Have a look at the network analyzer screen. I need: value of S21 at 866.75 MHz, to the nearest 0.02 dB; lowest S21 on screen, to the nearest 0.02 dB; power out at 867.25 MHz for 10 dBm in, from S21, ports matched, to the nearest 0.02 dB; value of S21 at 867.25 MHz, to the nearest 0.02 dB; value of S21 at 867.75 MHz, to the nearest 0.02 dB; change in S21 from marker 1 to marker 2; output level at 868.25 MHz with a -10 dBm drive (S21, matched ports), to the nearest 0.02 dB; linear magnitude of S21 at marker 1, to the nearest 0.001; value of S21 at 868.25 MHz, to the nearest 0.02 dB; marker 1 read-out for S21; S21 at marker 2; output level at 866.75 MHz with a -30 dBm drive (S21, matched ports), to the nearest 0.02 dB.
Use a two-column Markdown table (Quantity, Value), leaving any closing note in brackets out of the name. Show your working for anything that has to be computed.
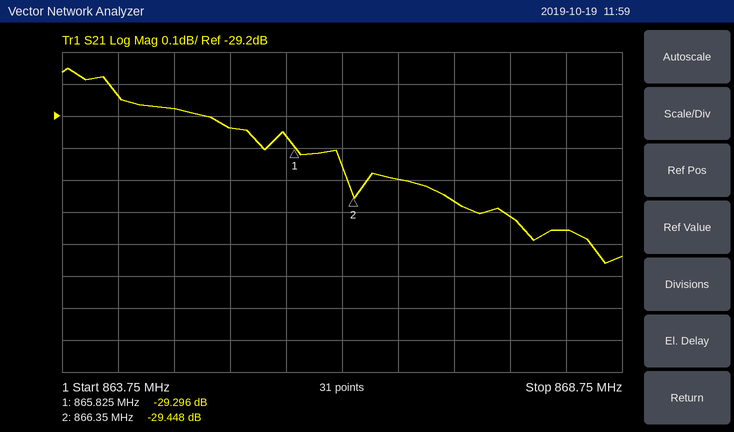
| Quantity | Value |
|---|---|
| value of S21 at 866.75 MHz, to the nearest 0.02 dB | -29.40 dB |
| lowest S21 on screen, to the nearest 0.02 dB | -29.66 dB |
| power out at 867.25 MHz for 10 dBm in, from S21, ports matched, to the nearest 0.02 dB | 10 dBm + (-29.46 dB) = -19.46 dBm |
| value of S21 at 867.25 MHz, to the nearest 0.02 dB | -29.46 dB |
| value of S21 at 867.75 MHz, to the nearest 0.02 dB | -29.52 dB |
| change in S21 from marker 1 to marker 2 | -29.448 − (-29.296) = -0.152 dB |
| output level at 868.25 MHz with a -10 dBm drive (S21, matched ports), to the nearest 0.02 dB | -10 dBm + (-29.56 dB) = -39.56 dBm |
| linear magnitude of S21 at marker 1, to the nearest 0.001 | 10^(-29.296/20) ≈ 0.034 |
| value of S21 at 868.25 MHz, to the nearest 0.02 dB | -29.56 dB |
| marker 1 read-out for S21 | -29.296 dB |
| S21 at marker 2 | -29.448 dB |
| output level at 866.75 MHz with a -30 dBm drive (S21, matched ports), to the nearest 0.02 dB | -30 dBm + (-29.40 dB) = -59.40 dBm |
